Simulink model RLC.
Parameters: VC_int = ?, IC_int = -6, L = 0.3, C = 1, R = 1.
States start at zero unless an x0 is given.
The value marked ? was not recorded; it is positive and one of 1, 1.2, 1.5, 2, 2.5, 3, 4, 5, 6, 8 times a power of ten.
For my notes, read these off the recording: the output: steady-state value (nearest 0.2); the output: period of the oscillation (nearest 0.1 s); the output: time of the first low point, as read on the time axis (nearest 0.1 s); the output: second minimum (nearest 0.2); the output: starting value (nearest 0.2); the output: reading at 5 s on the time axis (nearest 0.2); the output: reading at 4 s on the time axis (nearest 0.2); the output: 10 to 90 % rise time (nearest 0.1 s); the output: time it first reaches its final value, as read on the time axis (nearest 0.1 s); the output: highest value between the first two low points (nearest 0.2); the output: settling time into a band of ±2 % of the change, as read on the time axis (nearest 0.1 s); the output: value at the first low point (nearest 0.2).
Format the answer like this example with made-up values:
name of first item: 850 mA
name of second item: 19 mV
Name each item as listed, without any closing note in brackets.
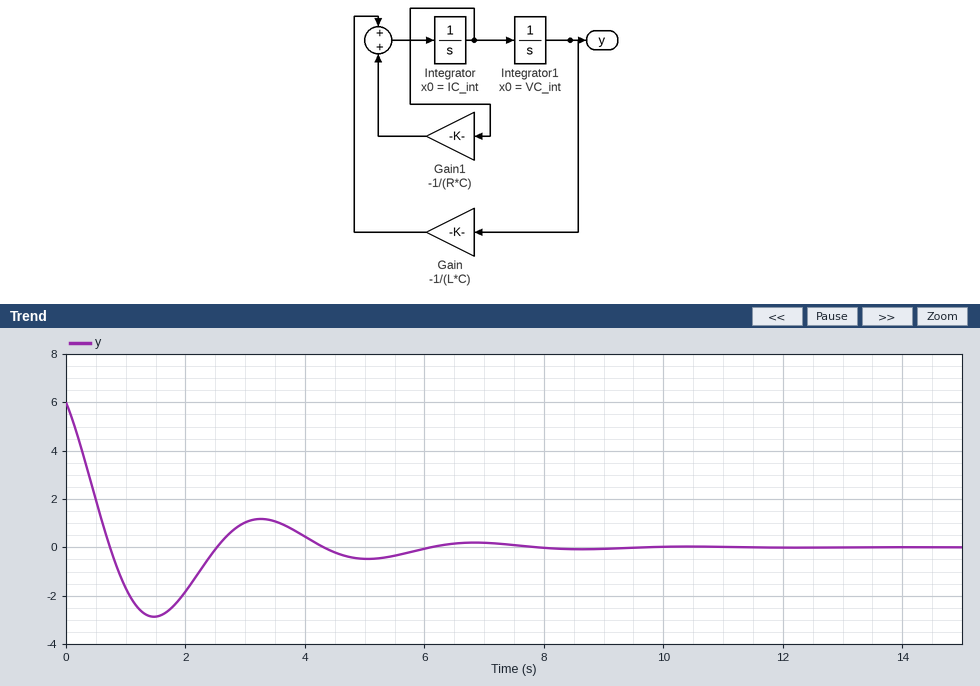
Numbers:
the output: steady-state value: 0.0
the output: period of the oscillation: 3.6 s
the output: time of the first low point, as read on the time axis: 1.5 s
the output: second minimum: -0.4
the output: starting value: 6.0
the output: reading at 5 s on the time axis: -0.4
the output: reading at 4 s on the time axis: 0.4
the output: 10 to 90 % rise time: 0.6 s
the output: time it first reaches its final value, as read on the time axis: 0.7 s
the output: highest value between the first two low points: 1.2
the output: settling time into a band of ±2 % of the change, as read on the time axis: 7.4 s
the output: value at the first low point: -2.8
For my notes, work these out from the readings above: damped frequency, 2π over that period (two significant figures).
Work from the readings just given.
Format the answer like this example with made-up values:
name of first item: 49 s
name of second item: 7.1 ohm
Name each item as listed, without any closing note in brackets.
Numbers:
damped frequency, 2π over that period: 1.7 rad/s
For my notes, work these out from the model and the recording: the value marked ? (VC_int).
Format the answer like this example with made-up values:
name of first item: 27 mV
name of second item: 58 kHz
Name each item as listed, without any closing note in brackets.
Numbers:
the value marked ?: 6
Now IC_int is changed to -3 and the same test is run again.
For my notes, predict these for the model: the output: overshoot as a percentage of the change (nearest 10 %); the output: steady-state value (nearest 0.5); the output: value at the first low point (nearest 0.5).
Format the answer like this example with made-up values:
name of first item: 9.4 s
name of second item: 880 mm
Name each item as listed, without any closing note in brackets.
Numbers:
the output: overshoot as a percentage of the change: 40 %
the output: steady-state value: 0.0
the output: value at the first low point: -2.5
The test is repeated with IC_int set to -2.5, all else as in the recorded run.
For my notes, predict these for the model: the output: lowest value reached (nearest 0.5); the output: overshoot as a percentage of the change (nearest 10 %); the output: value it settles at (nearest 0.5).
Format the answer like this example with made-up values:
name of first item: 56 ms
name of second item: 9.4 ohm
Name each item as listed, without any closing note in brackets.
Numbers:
the output: lowest value reached: -2.5
the output: overshoot as a percentage of the change: 40 %
the output: value it settles at: 0.0
